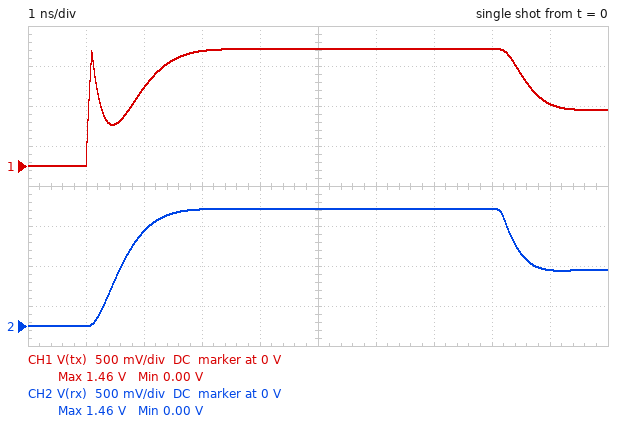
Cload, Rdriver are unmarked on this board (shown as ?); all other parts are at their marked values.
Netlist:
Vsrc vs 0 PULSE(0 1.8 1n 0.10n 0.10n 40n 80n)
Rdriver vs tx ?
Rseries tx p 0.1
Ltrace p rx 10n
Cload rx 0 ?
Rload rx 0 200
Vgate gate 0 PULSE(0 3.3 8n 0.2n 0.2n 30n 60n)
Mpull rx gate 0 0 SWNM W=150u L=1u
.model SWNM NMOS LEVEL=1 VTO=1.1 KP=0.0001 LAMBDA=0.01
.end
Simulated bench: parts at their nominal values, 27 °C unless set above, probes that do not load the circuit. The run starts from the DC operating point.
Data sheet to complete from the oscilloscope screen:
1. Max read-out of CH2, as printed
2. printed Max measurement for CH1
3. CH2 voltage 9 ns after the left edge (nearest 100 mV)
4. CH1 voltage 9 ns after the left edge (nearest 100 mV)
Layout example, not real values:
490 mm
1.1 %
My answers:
1.46 V
1.46 V
700 mV
800 mV
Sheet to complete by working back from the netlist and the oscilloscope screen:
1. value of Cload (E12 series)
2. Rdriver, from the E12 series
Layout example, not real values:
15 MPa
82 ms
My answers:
15 pF
47 Ω
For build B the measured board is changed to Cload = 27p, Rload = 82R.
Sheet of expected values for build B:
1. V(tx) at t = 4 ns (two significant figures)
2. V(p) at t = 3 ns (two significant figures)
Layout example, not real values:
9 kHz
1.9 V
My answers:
1.1 V
1.0 V
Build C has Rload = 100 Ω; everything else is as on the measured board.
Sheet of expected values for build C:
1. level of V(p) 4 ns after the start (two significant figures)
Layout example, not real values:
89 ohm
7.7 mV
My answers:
1.2 V
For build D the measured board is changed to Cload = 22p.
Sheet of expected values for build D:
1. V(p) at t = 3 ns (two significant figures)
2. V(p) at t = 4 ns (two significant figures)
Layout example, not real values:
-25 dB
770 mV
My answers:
1.3 V
1.4 V
